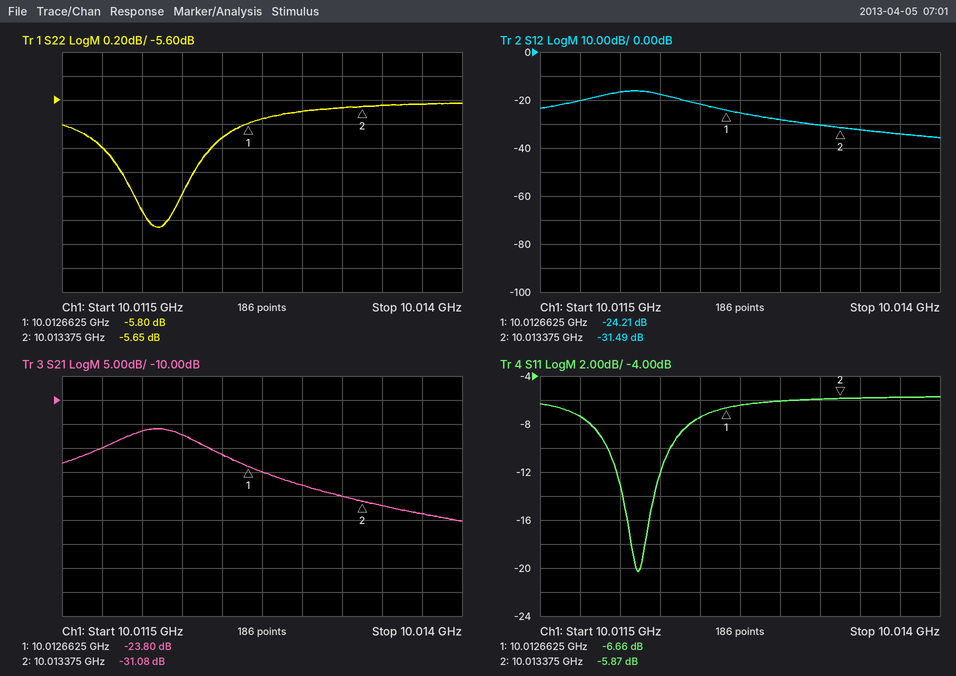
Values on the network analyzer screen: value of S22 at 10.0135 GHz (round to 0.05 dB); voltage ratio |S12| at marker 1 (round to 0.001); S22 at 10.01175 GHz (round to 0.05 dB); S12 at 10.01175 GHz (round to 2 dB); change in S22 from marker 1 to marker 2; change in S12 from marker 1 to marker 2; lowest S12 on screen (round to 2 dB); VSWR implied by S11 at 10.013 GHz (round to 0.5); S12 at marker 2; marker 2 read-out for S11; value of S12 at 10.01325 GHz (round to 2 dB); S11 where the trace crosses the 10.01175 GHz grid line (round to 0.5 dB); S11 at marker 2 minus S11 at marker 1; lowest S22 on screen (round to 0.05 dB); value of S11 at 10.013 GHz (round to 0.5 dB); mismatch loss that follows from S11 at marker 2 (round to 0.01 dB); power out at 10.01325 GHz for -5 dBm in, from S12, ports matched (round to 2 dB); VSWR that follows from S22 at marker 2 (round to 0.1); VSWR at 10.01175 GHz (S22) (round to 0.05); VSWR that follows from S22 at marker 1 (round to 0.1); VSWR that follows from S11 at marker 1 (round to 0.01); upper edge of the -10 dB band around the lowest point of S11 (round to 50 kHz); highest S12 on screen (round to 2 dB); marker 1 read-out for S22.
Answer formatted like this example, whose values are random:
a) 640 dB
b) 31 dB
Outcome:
a) -5.65 dB
b) 0.062
c) -6.00 dB
d) -20 dB
e) 0.15 dB
f) -7.28 dB
g) -36 dB
h) 3.0
i) -31.49 dB
j) -5.87 dB
k) -30 dB
l) -7.5 dB
m) 0.79 dB
n) -6.65 dB
o) -6.0 dB
p) 1.30 dB
q) -36 dBm
r) 3.2
s) 3.00
t) 3.1
u) 2.73
v) 10.01230 GHz
w) -16 dB
x) -5.80 dB
